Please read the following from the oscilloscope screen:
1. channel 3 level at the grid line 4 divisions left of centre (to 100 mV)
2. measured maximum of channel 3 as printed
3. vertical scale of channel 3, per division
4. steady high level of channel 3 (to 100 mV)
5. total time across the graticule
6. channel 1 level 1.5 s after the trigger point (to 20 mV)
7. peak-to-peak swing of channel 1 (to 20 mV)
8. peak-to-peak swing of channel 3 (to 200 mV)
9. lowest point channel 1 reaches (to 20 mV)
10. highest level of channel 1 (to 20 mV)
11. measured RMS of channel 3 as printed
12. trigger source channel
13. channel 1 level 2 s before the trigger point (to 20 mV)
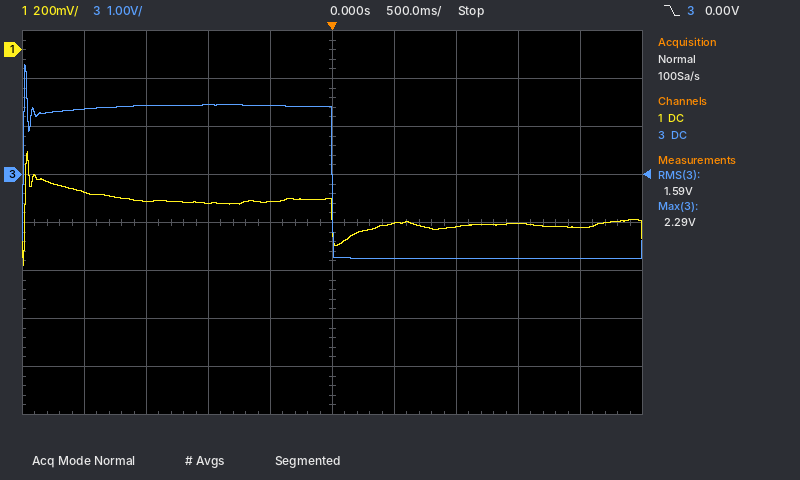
1.4 V
2.29 V
1 V
1.4 V
5 s
-720 mV
480 mV
4.0 V
-900 mV
-420 mV
1.59 V
channel 3
-600 mV
